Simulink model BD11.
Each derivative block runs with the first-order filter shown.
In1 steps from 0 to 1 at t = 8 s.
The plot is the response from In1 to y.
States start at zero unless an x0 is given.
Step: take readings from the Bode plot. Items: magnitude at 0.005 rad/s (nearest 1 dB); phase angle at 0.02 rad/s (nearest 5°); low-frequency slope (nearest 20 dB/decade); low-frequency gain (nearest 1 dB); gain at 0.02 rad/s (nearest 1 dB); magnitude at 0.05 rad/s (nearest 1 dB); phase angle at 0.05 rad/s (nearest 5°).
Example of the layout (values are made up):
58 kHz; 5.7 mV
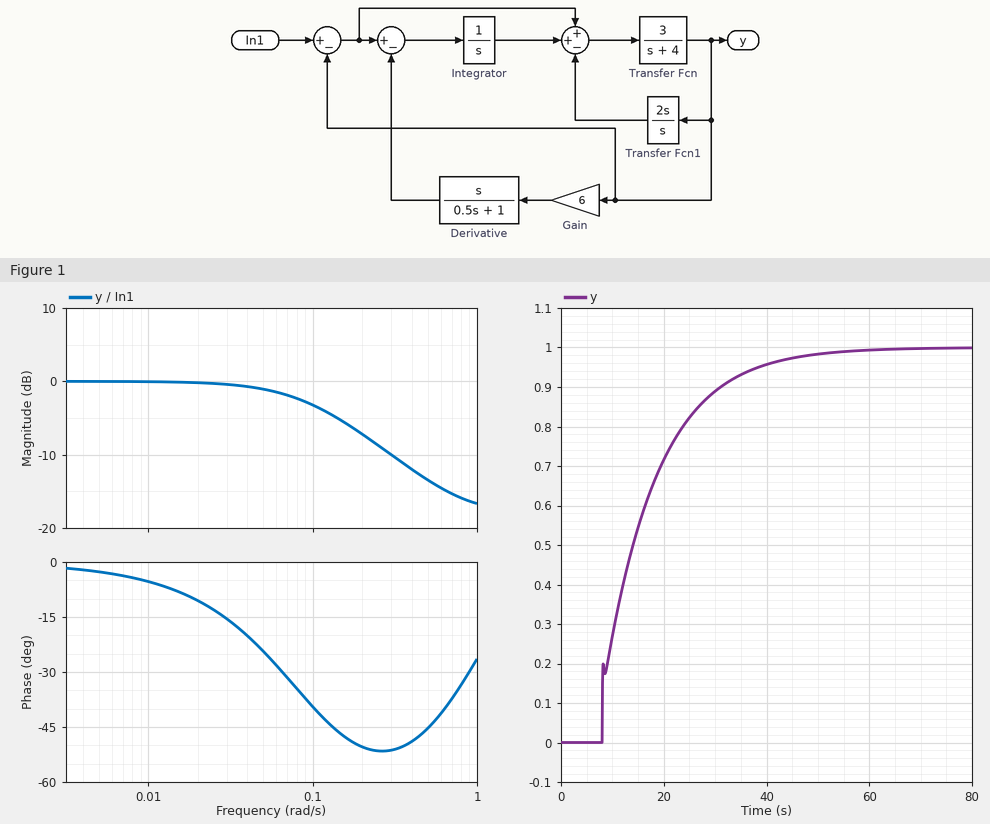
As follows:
0 dB; -10°; 0 dB/decade; 0 dB; 0 dB; -1 dB; -25°
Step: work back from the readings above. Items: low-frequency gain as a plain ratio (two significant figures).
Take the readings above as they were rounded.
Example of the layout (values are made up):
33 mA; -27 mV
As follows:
1.0
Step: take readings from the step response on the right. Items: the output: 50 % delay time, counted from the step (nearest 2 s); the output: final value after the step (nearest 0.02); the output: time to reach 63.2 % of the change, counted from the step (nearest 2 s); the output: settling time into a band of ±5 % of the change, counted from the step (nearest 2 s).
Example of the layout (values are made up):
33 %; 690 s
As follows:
6 s; 1.00; 10 s; 30 s
